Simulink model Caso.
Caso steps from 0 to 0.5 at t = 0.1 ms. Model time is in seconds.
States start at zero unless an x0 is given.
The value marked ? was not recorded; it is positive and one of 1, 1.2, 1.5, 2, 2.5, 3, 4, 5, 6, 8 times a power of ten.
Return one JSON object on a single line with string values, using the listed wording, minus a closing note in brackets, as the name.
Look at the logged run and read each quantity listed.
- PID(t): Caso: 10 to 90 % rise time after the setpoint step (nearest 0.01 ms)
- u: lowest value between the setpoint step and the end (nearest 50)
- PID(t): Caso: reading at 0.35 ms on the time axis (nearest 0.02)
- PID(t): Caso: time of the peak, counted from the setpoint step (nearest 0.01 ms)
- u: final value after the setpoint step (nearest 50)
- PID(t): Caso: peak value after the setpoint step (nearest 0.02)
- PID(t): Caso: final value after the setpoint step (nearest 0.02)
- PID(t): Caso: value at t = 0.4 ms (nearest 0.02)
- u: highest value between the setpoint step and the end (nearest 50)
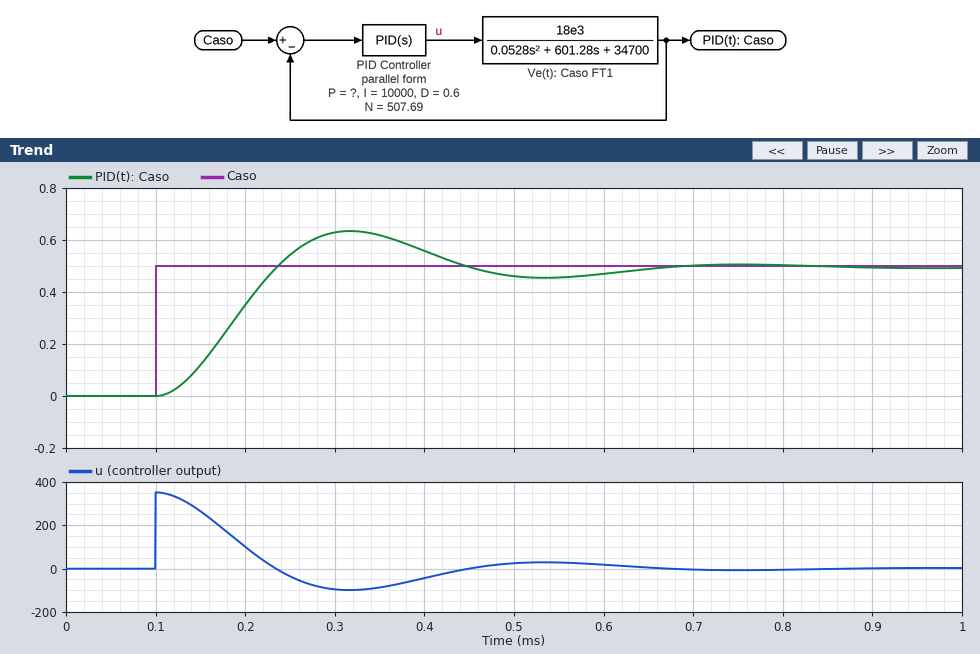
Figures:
{"PID(t): Caso: 10 to 90 % rise time after the setpoint step": "0.09 ms", "u: lowest value between the setpoint step and the end": "-100", "PID(t): Caso: reading at 0.35 ms on the time axis": "0.62", "PID(t): Caso: time of the peak, counted from the setpoint step": "0.22 ms", "u: final value after the setpoint step": "0", "PID(t): Caso: peak value after the setpoint step": "0.64", "PID(t): Caso: final value after the setpoint step": "0.50", "PID(t): Caso: value at t = 0.4 ms": "0.56", "u: highest value between the setpoint step and the end": "350"}
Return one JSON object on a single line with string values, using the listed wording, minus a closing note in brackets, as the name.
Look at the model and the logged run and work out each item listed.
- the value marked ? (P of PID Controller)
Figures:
{"the value marked ?": "400"}
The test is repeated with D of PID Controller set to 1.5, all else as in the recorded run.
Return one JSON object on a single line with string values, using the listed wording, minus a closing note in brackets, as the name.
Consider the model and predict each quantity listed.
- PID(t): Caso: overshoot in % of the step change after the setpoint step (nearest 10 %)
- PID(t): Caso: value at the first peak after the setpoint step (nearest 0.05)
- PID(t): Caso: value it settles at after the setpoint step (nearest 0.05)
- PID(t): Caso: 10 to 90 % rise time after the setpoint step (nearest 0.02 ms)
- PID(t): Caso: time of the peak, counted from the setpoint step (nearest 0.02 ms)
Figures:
{"PID(t): Caso: overshoot in % of the step change after the setpoint step": "40 %", "PID(t): Caso: value at the first peak after the setpoint step": "0.70", "PID(t): Caso: value it settles at after the setpoint step": "0.50", "PID(t): Caso: 10 to 90 % rise time after the setpoint step": "0.06 ms", "PID(t): Caso: time of the peak, counted from the setpoint step": "0.16 ms"}
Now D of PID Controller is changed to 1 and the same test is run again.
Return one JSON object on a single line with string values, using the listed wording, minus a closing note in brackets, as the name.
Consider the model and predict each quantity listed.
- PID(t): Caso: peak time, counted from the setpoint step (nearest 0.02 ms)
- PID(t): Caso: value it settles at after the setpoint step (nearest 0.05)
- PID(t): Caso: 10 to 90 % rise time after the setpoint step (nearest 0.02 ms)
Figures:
{"PID(t): Caso: peak time, counted from the setpoint step": "0.18 ms", "PID(t): Caso: value it settles at after the setpoint step": "0.50", "PID(t): Caso: 10 to 90 % rise time after the setpoint step": "0.08 ms"}
